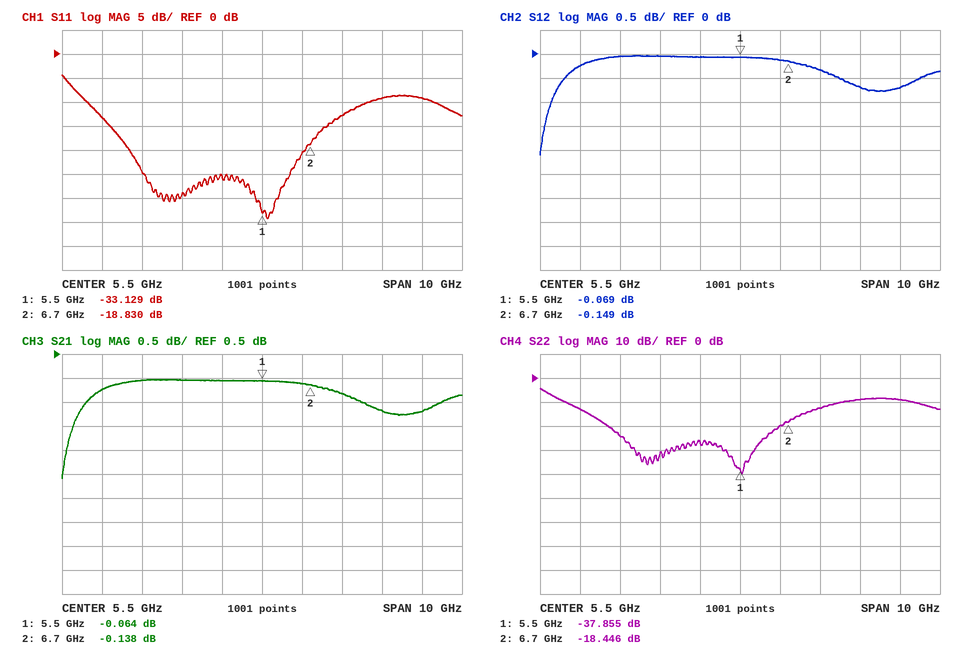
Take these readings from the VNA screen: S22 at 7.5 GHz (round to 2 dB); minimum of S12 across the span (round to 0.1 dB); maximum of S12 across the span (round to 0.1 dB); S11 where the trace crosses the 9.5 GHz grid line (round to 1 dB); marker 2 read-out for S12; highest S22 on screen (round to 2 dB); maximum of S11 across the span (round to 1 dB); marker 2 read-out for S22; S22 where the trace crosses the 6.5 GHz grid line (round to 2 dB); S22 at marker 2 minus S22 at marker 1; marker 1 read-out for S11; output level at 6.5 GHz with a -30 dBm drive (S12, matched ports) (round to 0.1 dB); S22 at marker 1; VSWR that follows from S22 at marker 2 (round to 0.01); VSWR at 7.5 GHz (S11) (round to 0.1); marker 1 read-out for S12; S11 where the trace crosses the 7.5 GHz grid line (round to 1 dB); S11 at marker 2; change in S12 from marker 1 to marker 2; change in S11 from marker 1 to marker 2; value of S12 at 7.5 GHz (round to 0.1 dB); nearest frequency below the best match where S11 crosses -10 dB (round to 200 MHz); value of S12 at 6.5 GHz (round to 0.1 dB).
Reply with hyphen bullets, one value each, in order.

- -12 dB
- -2.1 dB
- 0.0 dB
- -9 dB
- -0.149 dB
- -4 dB
- -4 dB
- -18.446 dB
- -20 dB
- 19.409 dB
- -33.129 dB
- -30.1 dBm
- -37.855 dB
- 1.27
- 1.6
- -0.069 dB
- -13 dB
- -18.830 dB
- -0.080 dB
- 14.299 dB
- -0.3 dB
- 1.2 GHz
- -0.1 dB
